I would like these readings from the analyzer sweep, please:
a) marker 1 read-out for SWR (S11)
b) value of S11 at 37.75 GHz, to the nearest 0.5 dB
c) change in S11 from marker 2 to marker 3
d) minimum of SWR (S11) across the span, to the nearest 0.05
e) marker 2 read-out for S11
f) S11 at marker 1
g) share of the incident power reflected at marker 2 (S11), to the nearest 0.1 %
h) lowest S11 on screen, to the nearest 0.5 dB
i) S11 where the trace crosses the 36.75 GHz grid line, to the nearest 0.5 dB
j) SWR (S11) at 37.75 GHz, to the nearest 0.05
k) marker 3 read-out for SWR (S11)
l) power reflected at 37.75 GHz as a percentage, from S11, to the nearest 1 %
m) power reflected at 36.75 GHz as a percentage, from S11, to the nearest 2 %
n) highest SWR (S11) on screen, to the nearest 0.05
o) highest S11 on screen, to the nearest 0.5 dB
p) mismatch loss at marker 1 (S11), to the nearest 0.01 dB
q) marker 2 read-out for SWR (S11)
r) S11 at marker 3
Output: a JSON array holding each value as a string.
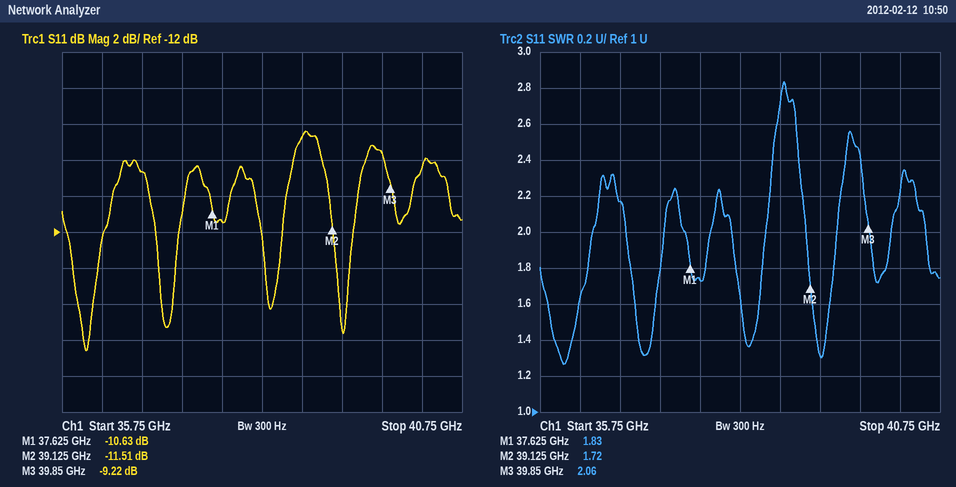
["1.83", "-11.5 dB", "2.29 dB", "1.25", "-11.51 dB", "-10.63 dB", "7.1 %", "-18.5 dB", "-8.5 dB", "1.75", "2.06", "7 %", "14 %", "2.85", "-6.5 dB", "0.39 dB", "1.72", "-9.22 dB"]
